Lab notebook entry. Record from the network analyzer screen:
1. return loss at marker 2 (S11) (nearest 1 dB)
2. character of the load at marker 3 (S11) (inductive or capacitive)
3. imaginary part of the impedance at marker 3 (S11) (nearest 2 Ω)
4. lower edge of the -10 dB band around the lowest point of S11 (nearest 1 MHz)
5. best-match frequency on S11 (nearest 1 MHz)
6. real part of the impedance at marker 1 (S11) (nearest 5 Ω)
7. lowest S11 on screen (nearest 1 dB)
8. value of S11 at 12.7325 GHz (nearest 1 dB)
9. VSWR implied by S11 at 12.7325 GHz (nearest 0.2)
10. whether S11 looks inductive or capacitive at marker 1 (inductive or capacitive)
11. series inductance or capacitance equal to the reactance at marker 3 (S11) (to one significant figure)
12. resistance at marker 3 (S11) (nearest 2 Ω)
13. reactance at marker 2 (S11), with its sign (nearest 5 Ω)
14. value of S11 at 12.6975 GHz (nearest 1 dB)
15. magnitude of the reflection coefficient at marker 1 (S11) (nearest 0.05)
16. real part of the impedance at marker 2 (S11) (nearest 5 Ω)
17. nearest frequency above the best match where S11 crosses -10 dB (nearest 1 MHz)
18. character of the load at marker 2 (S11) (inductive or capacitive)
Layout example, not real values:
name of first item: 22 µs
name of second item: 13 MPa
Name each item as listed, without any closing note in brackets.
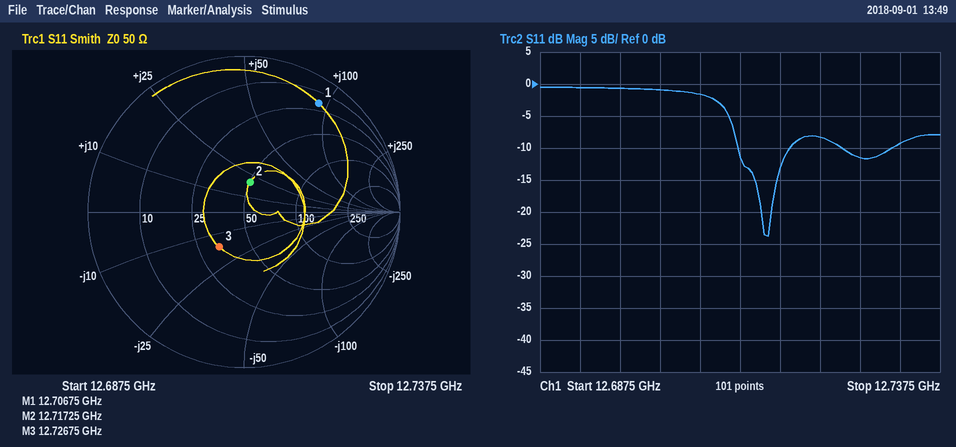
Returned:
return loss at marker 2 (S11): 14 dB
character of the load at marker 3 (S11): capacitive
imaginary part of the impedance at marker 3 (S11): -16 Ω
lower edge of the -10 dB band around the lowest point of S11: 12.712 GHz
best-match frequency on S11: 12.716 GHz
real part of the impedance at marker 1 (S11): 20 Ω
lowest S11 on screen: -24 dB
value of S11 at 12.7325 GHz: -9 dB
VSWR implied by S11 at 12.7325 GHz: 2.0
whether S11 looks inductive or capacitive at marker 1: inductive
series inductance or capacitance equal to the reactance at marker 3 (S11): 800 fF
resistance at marker 3 (S11): 34 Ω
reactance at marker 2 (S11), with its sign: +20 Ω
value of S11 at 12.6975 GHz: -1 dB
magnitude of the reflection coefficient at marker 1 (S11): 0.85
real part of the impedance at marker 2 (S11): 50 Ω
nearest frequency above the best match where S11 crosses -10 dB: 12.719 GHz
character of the load at marker 2 (S11): inductive
